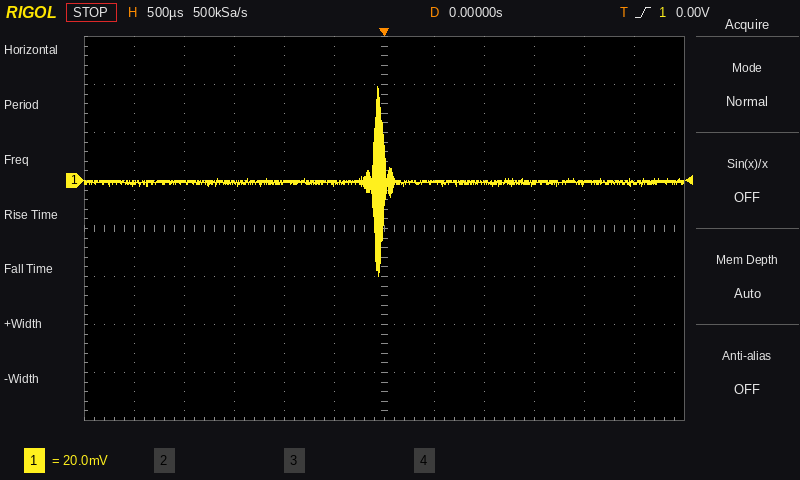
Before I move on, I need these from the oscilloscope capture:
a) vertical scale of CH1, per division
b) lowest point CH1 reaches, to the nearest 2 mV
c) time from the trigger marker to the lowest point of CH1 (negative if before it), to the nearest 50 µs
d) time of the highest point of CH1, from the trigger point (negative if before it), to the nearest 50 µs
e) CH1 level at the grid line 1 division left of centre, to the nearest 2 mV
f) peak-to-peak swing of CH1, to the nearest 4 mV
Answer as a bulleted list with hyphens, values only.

- 20 mV
- -40 mV
- -50 µs
- -50 µs
- -2 mV
- 80 mV
